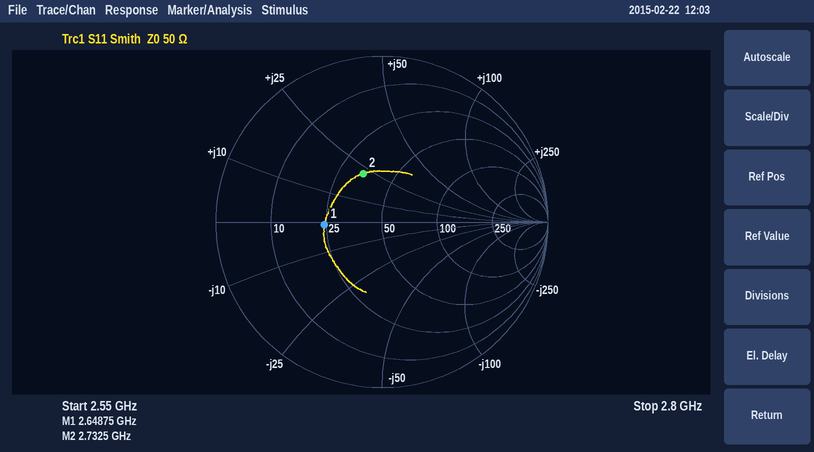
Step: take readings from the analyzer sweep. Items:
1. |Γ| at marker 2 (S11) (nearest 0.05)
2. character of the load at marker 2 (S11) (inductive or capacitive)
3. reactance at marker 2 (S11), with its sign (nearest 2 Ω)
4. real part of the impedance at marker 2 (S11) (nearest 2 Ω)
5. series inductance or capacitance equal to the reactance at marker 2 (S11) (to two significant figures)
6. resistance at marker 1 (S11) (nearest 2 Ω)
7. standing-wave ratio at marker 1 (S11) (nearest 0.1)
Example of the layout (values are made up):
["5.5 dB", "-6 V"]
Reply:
["0.30", "inductive", "+22 Ω", "34 Ω", "1.3 nH", "24 Ω", "2.1"]
